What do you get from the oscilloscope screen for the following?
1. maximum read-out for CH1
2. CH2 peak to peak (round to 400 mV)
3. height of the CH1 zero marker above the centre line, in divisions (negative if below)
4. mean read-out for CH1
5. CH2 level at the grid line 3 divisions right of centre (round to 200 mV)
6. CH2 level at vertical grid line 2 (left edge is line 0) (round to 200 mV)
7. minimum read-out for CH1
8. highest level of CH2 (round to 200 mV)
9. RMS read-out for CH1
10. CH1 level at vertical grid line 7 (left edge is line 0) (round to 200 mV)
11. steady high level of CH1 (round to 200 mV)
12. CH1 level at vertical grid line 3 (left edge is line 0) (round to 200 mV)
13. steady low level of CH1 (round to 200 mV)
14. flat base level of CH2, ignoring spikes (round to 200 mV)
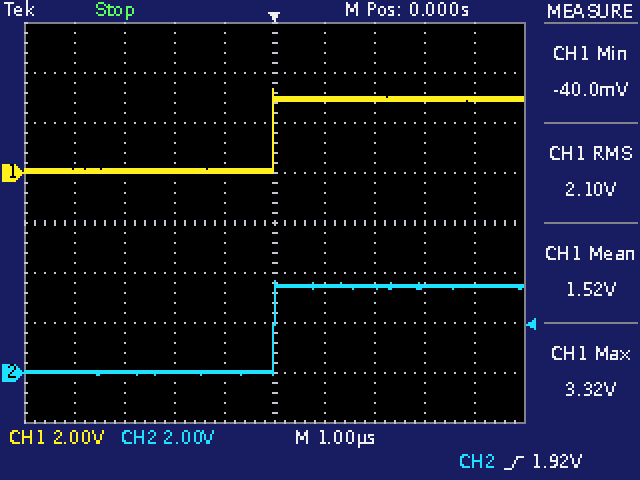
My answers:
3.32 V
3.6 V
+1.0 div
1.52 V
3.4 V
0.0 V
-40.0 mV
3.6 V
2.10 V
3.0 V
3.0 V
0.0 V
0.0 V
0.0 V
